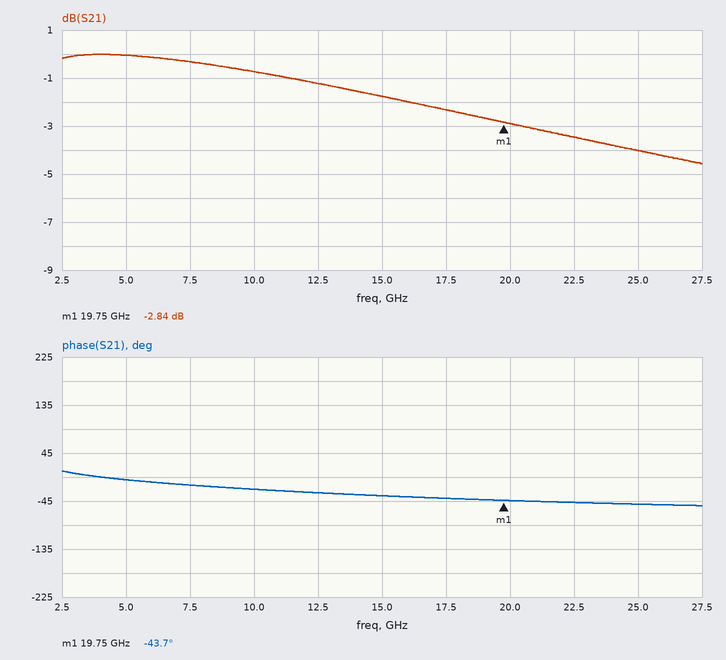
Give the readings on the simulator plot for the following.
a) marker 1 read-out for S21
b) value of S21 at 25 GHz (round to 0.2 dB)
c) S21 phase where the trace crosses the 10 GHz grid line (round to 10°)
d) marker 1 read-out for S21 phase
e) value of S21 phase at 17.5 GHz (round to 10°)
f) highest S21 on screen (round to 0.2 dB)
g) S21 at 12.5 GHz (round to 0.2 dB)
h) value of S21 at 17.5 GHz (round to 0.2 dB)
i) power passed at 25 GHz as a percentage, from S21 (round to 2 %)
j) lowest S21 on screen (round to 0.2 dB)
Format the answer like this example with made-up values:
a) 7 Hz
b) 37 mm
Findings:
a) -2.84 dB
b) -4.0 dB
c) -20°
d) -43.7°
e) -40°
f) 0.0 dB
g) -1.2 dB
h) -2.4 dB
i) 40 %
j) -4.6 dB
